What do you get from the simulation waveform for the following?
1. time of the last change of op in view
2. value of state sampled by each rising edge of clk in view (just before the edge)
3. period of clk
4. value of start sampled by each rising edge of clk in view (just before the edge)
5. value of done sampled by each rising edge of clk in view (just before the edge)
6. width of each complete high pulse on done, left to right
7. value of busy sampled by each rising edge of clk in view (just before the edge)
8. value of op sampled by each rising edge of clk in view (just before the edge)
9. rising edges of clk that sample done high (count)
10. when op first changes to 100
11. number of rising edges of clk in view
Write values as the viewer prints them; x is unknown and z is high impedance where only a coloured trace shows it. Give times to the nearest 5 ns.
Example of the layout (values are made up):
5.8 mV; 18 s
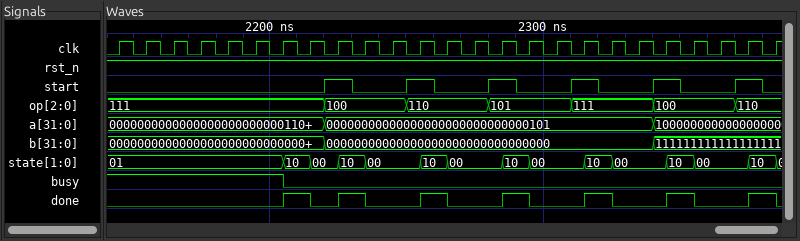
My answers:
2370 ns; 01, 01, 01, 01, 01, 01, 01, 10, 00, 10, 00, 00, 10, 00, 00, 10, 00, 00, 10, 00, 00, 10, 00, 00, 10; 10 ns; 0 0 0 0 0 0 0 0 1 0 0 1 0 0 1 0 0 1 0 0 1 0 0 1 0; 0 0 0 0 0 0 0 1 0 1 0 0 1 0 0 1 0 0 1 0 0 1 0 0 1; 10 ns, 10 ns, 10 ns, 10 ns, 10 ns, 10 ns, 10 ns; 1 1 1 1 1 1 1 0 0 0 0 0 0 0 0 0 0 0 0 0 0 0 0 0 0; 111, 111, 111, 111, 111, 111, 111, 111, 100, 100, 100, 110, 110, 110, 101, 101, 101, 111, 111, 111, 100, 100, 100, 110, 110; 7; 2220 ns; 25
